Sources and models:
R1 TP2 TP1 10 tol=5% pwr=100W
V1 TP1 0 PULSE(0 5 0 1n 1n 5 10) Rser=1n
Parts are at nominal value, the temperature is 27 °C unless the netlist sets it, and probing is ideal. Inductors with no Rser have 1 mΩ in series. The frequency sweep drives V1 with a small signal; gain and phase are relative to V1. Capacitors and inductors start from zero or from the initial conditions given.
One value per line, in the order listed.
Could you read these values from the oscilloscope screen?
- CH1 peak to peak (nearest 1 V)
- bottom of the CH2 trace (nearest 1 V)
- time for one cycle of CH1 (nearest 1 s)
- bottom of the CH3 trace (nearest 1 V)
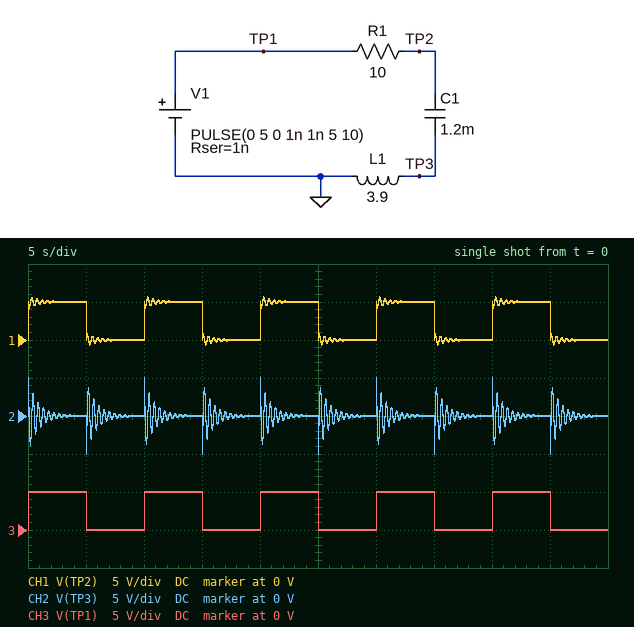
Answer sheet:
6 V
-5 V
10 s
0 V
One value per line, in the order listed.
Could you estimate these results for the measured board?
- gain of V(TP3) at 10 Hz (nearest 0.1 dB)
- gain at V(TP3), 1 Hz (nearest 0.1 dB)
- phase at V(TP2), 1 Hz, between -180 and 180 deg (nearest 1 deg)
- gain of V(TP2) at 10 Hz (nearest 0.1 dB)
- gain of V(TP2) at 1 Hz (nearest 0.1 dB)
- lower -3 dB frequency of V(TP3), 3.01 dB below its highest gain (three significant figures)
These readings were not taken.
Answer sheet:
0.5 dB
-12.9 dB
-5 deg
0 dB
0 dB
2.16 Hz
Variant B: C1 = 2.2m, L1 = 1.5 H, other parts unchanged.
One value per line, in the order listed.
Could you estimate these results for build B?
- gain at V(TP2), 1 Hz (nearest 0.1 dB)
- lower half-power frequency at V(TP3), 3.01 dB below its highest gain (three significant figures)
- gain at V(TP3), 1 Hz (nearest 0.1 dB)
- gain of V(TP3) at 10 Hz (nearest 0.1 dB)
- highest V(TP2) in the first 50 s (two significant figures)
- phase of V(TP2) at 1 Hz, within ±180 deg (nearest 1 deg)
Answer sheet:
-0.1 dB
2.43 Hz
-16.6 dB
0.6 dB
5.8 V
-9 deg
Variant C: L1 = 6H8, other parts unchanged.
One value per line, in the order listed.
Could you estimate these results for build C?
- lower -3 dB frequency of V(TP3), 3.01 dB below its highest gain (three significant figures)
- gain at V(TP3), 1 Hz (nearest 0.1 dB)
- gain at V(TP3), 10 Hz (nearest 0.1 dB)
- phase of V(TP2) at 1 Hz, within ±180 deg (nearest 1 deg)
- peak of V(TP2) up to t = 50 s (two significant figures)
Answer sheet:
1.66 Hz
-6.5 dB
0.3 dB
-6 deg
5.5 V
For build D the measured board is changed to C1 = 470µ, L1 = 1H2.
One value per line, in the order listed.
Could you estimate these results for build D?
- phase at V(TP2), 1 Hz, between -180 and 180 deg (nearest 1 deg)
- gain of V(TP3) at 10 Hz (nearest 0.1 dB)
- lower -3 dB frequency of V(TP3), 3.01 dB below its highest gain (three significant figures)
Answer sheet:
-2 deg
4.9 dB
6.18 Hz
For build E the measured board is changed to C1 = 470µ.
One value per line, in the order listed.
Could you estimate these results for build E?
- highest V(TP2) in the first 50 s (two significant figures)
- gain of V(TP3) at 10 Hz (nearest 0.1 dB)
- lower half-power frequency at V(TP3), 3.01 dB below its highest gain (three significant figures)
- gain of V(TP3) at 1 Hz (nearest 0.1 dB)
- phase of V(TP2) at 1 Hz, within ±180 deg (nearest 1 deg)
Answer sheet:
5.4 V
1.3 dB
3.54 Hz
-22.2 dB
-2 deg
